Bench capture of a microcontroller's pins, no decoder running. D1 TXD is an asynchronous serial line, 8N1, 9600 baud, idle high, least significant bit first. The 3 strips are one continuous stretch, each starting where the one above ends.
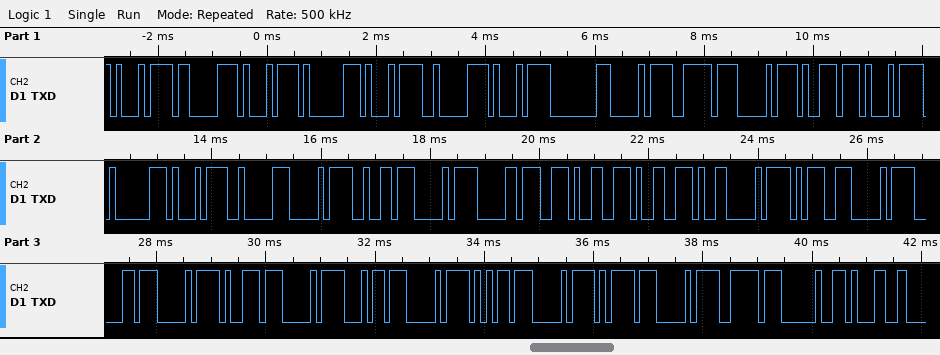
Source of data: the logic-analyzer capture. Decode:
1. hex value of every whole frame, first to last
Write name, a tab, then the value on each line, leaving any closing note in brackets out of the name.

hex value of every whole frame, first to last	D1 83 D1 81 D1 82 D1 80 D0 BE D0 B9 D1 81 D1 82 D0 B2 D0 B0 2E 2E 2E D0 9D D0 B0 D0 B9 D0 B4 D0 B5 D0 BD D0 BE 20 31
